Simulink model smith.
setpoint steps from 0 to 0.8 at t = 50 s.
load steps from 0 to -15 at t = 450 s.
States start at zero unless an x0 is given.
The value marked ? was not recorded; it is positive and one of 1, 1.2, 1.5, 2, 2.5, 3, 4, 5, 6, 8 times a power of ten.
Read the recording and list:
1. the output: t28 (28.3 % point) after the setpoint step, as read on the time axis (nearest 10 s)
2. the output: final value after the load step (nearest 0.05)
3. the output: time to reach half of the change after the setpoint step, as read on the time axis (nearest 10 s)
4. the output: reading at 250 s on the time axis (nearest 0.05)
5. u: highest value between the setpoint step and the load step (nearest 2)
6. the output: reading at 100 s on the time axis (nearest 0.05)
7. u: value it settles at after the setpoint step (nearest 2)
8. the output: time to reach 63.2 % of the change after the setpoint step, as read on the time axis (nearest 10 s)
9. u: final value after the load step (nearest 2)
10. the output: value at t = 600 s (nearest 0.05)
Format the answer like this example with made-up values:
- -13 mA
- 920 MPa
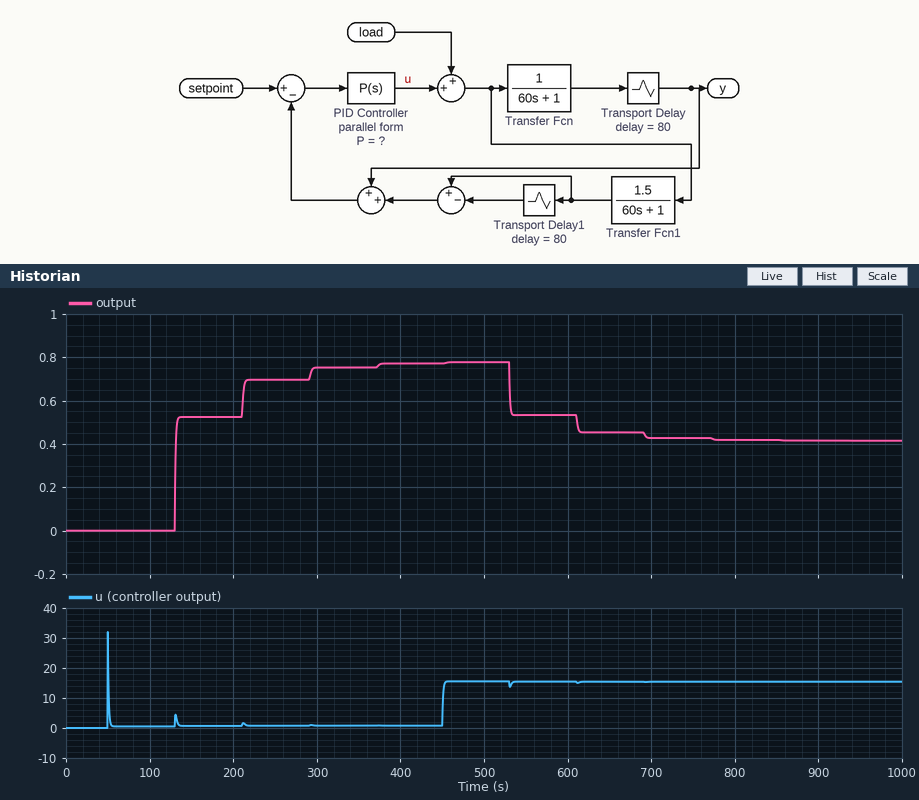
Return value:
- 130 s
- 0.40
- 130 s
- 0.70
- 32
- 0.00
- 0
- 130 s
- 16
- 0.55
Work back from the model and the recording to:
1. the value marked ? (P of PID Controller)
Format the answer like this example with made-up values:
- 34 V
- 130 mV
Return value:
- 40
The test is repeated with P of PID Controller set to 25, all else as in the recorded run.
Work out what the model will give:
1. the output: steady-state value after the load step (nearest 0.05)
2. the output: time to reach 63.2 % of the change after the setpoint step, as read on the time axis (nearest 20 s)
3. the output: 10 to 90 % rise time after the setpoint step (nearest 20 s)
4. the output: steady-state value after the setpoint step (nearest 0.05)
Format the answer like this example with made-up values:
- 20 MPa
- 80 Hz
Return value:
- 0.20
- 140 s
- 160 s
- 0.75
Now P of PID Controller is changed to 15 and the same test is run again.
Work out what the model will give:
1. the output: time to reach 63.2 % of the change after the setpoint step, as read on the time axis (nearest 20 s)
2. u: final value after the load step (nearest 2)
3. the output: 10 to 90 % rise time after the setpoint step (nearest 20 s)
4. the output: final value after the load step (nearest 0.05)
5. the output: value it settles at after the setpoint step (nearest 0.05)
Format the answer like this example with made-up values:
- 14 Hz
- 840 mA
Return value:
- 140 s
- 14
- 160 s
- -0.20
- 0.75
